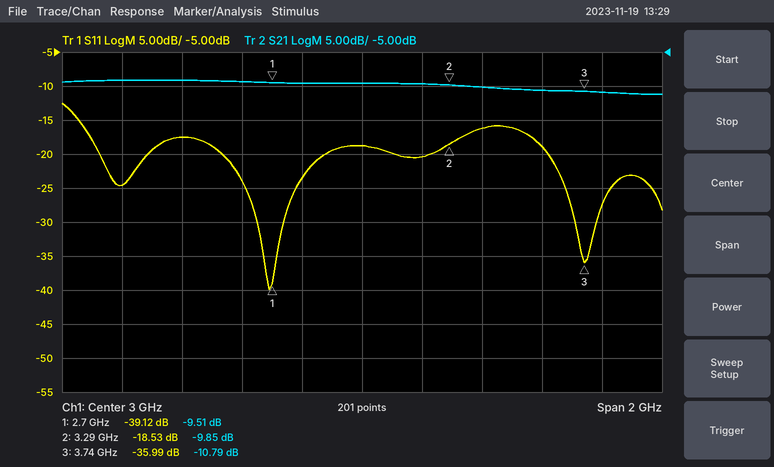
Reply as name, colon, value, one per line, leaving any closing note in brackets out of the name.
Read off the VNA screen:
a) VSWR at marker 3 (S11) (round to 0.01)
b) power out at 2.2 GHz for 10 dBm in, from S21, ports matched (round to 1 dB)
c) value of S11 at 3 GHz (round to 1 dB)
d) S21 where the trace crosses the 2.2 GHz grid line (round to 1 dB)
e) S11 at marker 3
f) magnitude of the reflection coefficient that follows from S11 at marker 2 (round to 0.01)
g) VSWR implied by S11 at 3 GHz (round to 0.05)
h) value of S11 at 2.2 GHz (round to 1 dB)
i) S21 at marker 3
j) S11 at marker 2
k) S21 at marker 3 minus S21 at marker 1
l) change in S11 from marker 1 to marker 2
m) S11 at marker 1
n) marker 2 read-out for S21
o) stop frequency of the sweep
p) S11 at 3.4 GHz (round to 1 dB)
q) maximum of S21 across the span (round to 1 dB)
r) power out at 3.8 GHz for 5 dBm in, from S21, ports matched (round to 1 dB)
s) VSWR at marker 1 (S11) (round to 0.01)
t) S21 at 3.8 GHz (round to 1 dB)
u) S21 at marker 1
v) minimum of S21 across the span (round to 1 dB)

VSWR at marker 3 (S11): 1.03
power out at 2.2 GHz for 10 dBm in, from S21, ports matched: 1 dBm
value of S11 at 3 GHz: -19 dB
S21 where the trace crosses the 2.2 GHz grid line: -9 dB
S11 at marker 3: -35.99 dB
magnitude of the reflection coefficient that follows from S11 at marker 2: 0.12
VSWR implied by S11 at 3 GHz: 1.25
value of S11 at 2.2 GHz: -25 dB
S21 at marker 3: -10.79 dB
S11 at marker 2: -18.53 dB
S21 at marker 3 minus S21 at marker 1: -1.28 dB
change in S11 from marker 1 to marker 2: 20.59 dB
S11 at marker 1: -39.12 dB
marker 2 read-out for S21: -9.85 dB
stop frequency of the sweep: 4 GHz
S11 at 3.4 GHz: -16 dB
maximum of S21 across the span: -9 dB
power out at 3.8 GHz for 5 dBm in, from S21, ports matched: -6 dBm
VSWR at marker 1 (S11): 1.02
S21 at 3.8 GHz: -11 dB
S21 at marker 1: -9.51 dB
minimum of S21 across the span: -11 dB
